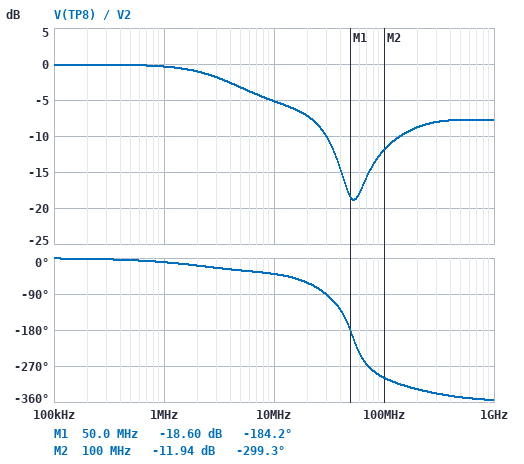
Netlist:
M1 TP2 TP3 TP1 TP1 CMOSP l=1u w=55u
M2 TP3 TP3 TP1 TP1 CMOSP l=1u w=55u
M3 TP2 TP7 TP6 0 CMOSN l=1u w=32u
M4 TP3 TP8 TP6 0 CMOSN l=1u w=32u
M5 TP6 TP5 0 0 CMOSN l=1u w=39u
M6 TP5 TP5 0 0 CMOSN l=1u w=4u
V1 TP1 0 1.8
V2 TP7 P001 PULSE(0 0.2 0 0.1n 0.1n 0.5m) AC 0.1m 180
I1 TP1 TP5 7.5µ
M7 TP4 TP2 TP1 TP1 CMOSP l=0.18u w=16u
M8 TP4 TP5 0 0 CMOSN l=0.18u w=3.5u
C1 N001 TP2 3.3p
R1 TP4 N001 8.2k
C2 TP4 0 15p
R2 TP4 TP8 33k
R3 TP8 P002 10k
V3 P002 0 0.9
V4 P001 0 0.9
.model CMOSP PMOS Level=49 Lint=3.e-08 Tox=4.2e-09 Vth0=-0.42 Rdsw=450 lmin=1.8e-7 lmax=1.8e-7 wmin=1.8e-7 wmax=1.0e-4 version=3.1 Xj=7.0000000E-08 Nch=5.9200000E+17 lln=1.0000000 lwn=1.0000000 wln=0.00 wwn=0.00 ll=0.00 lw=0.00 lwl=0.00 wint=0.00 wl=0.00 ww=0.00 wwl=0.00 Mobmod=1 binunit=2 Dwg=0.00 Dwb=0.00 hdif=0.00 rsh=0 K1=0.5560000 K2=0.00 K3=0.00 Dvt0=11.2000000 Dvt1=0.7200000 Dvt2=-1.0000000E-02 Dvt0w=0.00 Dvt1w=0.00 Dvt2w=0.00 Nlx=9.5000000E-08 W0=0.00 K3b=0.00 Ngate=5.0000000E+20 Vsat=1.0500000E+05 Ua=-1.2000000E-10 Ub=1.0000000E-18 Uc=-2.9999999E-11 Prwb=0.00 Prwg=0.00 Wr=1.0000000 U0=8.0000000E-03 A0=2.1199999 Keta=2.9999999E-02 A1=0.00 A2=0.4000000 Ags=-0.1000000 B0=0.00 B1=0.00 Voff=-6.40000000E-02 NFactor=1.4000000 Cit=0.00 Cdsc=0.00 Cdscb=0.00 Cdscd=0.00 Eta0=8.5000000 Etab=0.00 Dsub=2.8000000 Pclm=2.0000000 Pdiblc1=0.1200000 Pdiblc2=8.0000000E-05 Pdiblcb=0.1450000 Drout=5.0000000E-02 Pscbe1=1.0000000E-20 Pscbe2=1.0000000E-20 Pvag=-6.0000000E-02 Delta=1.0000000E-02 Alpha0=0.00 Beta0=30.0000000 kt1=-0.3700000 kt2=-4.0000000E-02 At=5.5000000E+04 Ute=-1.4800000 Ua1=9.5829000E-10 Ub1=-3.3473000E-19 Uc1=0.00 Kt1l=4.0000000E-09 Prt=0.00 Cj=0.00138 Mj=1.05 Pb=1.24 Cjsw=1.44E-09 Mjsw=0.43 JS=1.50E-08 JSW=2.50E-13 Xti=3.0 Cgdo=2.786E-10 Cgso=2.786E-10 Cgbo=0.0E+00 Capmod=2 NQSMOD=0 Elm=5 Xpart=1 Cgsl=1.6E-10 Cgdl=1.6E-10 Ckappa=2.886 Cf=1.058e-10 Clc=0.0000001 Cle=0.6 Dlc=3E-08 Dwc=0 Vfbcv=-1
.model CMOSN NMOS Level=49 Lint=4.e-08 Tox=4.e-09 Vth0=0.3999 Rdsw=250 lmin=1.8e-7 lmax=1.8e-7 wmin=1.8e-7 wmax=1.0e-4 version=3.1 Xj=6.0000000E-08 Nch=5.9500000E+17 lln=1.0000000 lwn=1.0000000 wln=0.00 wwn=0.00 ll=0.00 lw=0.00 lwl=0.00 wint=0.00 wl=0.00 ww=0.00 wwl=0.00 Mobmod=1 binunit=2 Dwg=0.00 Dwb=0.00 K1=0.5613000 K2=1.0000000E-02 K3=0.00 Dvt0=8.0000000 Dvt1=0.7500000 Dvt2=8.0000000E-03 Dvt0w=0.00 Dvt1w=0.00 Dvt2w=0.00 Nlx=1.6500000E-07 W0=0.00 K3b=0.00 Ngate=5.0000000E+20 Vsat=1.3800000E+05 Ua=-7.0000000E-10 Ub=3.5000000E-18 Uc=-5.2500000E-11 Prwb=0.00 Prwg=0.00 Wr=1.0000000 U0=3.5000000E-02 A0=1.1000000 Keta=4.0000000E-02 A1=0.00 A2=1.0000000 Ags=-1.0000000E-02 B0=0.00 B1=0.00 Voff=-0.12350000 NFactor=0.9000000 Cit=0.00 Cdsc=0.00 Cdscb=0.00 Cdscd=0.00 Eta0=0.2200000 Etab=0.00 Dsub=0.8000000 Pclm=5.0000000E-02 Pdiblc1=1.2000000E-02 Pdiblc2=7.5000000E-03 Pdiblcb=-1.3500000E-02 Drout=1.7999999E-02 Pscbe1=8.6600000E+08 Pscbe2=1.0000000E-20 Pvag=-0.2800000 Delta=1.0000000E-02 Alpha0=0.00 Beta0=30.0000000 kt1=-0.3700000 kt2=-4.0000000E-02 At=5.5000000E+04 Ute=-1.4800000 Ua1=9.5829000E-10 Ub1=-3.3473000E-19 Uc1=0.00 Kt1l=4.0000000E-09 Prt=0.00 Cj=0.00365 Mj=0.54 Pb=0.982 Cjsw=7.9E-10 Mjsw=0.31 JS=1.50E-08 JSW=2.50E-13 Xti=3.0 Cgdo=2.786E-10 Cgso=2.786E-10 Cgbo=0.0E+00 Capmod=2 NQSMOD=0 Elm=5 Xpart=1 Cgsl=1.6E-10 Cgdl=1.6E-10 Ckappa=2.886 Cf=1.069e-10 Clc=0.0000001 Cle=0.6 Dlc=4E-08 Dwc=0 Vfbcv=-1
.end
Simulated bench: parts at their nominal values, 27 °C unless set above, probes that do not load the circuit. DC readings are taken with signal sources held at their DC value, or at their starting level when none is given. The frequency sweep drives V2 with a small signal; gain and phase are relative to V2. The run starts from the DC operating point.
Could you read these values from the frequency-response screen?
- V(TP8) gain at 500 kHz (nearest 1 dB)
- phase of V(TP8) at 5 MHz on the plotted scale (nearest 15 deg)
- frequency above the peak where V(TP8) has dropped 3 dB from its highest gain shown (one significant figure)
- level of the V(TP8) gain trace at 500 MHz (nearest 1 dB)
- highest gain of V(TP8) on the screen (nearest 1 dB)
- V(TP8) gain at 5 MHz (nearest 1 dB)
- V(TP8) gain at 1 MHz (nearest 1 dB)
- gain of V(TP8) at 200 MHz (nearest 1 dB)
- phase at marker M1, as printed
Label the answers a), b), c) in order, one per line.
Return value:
a) 0 dB
b) -30 deg
c) 5 MHz
d) -8 dB
e) 0 dB
f) -3 dB
g) 0 dB
h) -9 dB
i) -184.2 deg
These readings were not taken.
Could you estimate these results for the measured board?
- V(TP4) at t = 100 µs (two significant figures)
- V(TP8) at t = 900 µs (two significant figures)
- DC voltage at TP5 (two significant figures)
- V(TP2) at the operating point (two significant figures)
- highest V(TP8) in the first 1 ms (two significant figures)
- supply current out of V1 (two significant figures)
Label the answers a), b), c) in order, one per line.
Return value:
a) 1.7 V
b) 900 mV
c) 540 mV
d) 1.4 V
e) 1.1 V
f) 200 µA
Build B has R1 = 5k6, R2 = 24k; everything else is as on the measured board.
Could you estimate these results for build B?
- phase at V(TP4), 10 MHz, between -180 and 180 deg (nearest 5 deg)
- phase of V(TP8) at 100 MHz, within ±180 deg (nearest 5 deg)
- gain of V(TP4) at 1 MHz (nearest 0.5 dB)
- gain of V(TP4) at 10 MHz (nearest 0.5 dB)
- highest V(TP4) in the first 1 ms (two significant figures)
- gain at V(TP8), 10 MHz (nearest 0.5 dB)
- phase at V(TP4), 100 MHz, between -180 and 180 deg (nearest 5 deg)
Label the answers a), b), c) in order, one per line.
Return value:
a) -45 deg
b) 65 deg
c) 10.5 dB
d) 6.5 dB
e) 1.6 V
f) -4.5 dB
g) -155 deg
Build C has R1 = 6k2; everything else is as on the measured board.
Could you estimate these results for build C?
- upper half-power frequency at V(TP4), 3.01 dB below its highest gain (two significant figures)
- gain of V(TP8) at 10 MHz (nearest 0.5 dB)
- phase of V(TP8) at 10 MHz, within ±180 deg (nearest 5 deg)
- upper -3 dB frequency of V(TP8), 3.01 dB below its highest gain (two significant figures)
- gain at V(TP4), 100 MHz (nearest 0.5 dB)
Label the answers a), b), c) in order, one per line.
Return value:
a) 5.1 MHz
b) -6.0 dB
c) -50 deg
d) 4.9 MHz
e) -13.0 dB
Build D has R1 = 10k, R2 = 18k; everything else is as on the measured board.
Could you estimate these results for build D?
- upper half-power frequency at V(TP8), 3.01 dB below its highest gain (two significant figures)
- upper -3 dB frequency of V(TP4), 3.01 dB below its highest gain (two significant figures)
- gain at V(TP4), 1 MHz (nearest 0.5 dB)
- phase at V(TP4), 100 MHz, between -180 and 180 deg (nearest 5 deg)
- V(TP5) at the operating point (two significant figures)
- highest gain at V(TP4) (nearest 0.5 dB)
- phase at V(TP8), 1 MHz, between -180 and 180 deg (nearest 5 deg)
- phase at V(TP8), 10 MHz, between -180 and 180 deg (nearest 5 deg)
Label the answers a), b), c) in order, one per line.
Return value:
a) 12 MHz
b) 37 MHz
c) 8.5 dB
d) -170 deg
e) 540 mV
f) 9.0 dB
g) -5 deg
h) -25 deg
